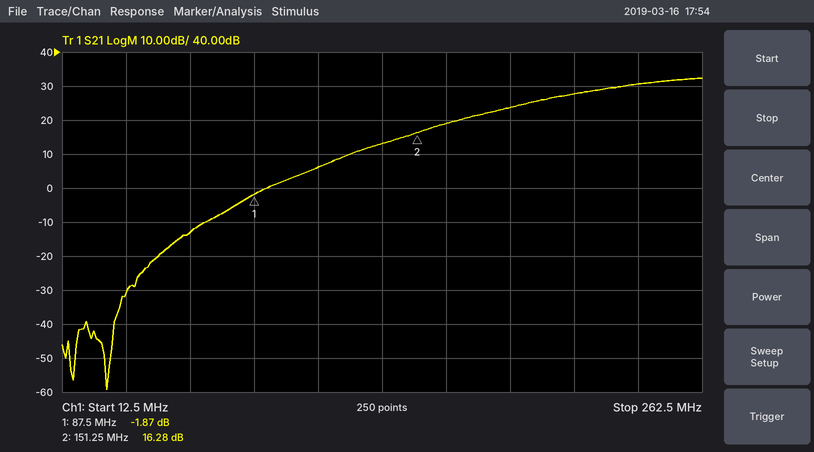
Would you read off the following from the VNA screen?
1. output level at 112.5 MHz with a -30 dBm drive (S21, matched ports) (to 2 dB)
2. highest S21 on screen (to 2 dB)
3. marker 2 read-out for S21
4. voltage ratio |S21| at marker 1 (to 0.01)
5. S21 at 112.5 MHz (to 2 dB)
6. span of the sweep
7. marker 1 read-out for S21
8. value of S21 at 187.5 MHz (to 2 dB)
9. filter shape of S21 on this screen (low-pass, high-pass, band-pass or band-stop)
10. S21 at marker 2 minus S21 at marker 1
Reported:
-24 dBm
32 dB
16.28 dB
0.81
6 dB
250 MHz
-1.87 dB
24 dB
high-pass
18.15 dB
